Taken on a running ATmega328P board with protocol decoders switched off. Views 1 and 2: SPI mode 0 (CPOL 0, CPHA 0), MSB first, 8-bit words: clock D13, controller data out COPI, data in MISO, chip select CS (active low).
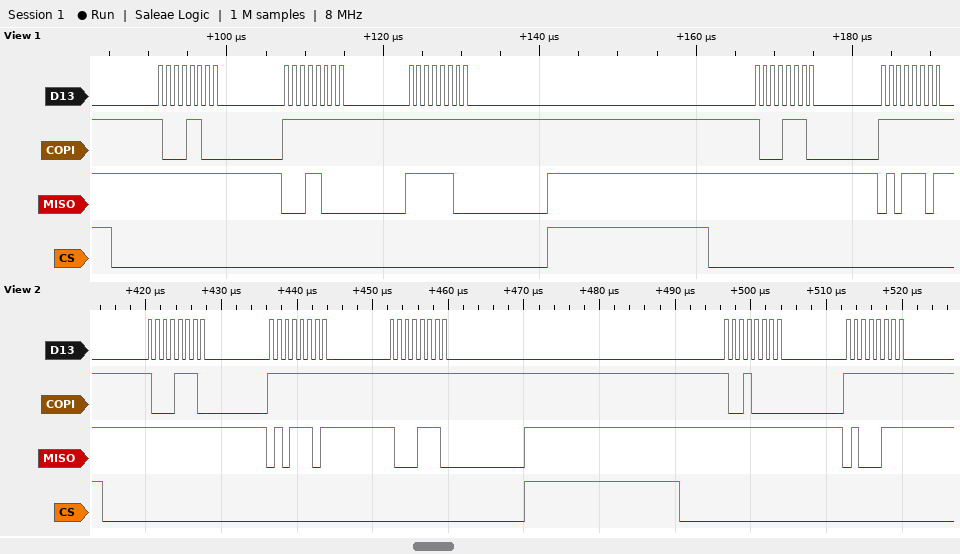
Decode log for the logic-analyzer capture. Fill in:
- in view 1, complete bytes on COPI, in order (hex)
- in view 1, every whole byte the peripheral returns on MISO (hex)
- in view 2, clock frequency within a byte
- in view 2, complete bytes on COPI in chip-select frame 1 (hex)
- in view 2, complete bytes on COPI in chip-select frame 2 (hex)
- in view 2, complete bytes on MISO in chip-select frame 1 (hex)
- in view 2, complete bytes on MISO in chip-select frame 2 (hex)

8C FF FF 8E FF
FF 18 FC FF 5D
1 MHz
8E FF FF
90 FF
FF 5D 8E
FF 47
